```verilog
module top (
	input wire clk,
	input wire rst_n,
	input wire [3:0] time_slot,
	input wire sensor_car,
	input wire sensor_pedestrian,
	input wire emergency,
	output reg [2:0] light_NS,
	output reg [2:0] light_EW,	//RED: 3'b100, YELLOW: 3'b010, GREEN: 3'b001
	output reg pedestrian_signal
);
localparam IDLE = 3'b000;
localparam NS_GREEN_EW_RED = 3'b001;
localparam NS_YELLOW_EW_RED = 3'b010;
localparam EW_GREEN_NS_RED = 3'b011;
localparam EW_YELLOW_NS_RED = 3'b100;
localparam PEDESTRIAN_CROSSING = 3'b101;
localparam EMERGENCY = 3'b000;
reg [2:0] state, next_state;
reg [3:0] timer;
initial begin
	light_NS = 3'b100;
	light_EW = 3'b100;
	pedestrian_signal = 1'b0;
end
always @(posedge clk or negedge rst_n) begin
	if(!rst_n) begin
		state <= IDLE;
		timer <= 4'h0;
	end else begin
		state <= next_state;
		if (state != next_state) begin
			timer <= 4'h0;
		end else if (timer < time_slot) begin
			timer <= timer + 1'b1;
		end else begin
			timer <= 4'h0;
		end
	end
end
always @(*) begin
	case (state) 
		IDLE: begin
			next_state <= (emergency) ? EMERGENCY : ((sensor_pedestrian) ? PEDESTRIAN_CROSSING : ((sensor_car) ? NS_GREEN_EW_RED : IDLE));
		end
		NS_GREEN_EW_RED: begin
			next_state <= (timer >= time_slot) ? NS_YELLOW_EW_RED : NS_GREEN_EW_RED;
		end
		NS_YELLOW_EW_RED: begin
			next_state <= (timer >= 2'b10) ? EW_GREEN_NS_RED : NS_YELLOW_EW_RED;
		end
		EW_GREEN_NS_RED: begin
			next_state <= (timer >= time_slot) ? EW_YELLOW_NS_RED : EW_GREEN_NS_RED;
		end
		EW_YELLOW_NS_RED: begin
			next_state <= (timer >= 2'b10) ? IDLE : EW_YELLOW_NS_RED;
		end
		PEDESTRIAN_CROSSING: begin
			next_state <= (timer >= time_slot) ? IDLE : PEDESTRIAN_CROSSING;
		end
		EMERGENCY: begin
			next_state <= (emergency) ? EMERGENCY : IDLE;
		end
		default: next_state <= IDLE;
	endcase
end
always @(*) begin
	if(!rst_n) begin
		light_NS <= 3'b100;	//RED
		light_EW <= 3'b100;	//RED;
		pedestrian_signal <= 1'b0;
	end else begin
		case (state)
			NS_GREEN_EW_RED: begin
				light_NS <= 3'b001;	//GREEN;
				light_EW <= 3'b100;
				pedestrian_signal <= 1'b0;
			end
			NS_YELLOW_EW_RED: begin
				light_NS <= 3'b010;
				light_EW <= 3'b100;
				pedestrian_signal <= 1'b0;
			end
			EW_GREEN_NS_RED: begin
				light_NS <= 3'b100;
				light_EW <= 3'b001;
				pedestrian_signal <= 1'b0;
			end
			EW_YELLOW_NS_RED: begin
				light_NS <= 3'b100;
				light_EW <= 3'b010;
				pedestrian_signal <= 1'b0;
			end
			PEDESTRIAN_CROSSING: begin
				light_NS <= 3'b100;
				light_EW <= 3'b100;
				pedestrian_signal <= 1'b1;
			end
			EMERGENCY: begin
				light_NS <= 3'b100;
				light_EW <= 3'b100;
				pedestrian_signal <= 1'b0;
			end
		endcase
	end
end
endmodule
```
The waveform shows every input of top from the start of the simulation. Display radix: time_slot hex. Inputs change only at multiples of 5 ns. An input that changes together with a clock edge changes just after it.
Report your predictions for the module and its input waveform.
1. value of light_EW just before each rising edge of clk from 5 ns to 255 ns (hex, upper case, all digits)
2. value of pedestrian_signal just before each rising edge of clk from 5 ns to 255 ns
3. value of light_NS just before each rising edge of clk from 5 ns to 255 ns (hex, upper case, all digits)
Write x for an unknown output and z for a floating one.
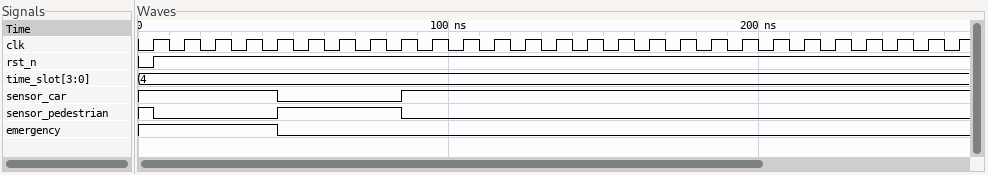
4, 4, 4, 4, 4, 4, 4, 4, 4, 4, 4, 4, 4, 4, 4, 4, 4, 4, 4, 4, 1, 1, 1, 1, 1, 2
0 0 0 0 0 0 1 1 1 1 1 0 0 0 0 0 0 0 0 0 0 0 0 0 0 0
4, 4, 4, 4, 4, 4, 4, 4, 4, 4, 4, 4, 1, 1, 1, 1, 1, 2, 2, 2, 4, 4, 4, 4, 4, 4
